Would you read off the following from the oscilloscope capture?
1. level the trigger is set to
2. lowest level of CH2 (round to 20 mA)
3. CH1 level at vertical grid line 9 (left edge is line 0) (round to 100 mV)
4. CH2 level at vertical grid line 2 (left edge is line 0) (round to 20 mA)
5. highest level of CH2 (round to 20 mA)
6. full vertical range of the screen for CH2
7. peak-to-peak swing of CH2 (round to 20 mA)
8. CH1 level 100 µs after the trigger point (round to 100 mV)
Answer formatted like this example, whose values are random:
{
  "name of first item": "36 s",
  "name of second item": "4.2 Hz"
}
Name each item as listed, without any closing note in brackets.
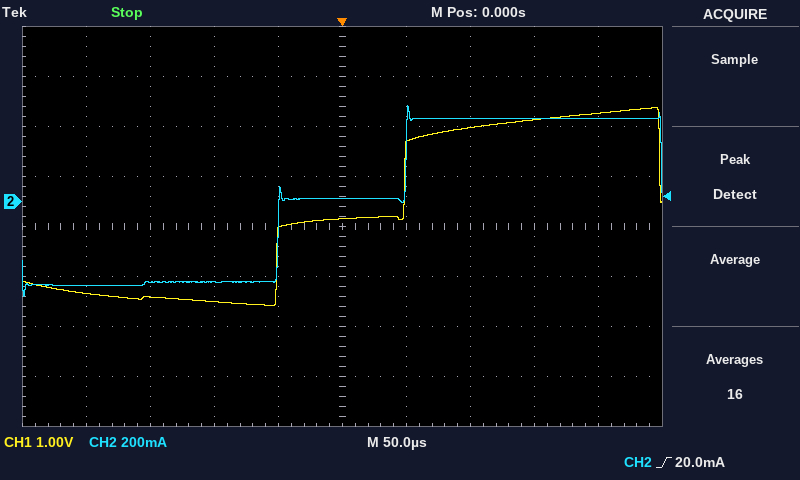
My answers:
{
  "level the trigger is set to": "20.0 mA",
  "lowest level of CH2": "-380 mA",
  "CH1 level at vertical grid line 9 (left edge is line 0)": "1.8 V",
  "CH2 level at vertical grid line 2 (left edge is line 0)": "-320 mA",
  "highest level of CH2": "380 mA",
  "full vertical range of the screen for CH2": "1.6 A",
  "peak-to-peak swing of CH2": "760 mA",
  "CH1 level 100 µs after the trigger point": "1.5 V"
}
